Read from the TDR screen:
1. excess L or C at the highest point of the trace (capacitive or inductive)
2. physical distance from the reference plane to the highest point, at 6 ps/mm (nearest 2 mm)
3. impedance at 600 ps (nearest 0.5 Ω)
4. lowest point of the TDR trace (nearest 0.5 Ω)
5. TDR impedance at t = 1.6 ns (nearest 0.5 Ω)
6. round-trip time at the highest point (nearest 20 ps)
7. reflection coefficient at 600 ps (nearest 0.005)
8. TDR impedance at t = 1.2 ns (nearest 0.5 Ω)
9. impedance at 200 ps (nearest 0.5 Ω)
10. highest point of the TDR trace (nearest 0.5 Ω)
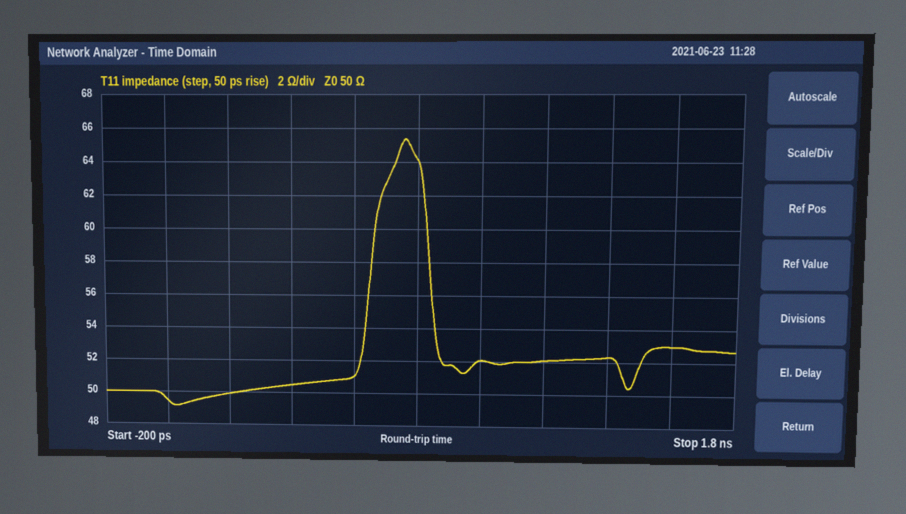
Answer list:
inductive
64 mm
51.0 Ω
49.0 Ω
53.0 Ω
760 ps
+0.010
52.0 Ω
50.0 Ω
65.5 Ω
